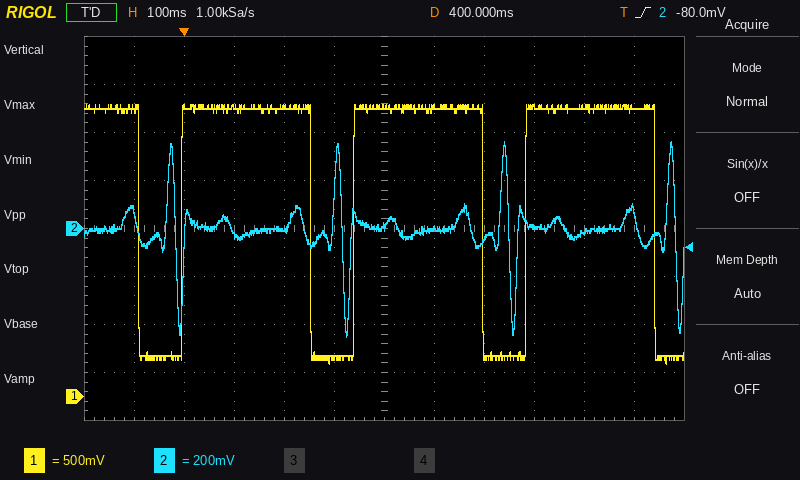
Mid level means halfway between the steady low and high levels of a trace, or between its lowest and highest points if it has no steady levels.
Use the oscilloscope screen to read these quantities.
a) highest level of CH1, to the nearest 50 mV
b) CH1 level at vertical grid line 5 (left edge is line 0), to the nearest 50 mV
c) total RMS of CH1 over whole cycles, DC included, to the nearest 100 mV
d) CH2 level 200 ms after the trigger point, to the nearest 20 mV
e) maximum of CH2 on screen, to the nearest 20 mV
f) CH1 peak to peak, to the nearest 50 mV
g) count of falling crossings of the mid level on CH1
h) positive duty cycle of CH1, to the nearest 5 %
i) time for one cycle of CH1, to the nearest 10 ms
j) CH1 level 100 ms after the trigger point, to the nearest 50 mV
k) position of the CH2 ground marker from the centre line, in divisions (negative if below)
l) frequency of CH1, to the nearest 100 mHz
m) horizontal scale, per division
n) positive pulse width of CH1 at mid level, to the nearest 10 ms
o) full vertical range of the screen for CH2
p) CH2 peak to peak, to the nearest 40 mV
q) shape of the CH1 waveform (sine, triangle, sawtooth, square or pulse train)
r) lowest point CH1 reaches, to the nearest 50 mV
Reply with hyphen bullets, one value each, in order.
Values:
- 3.05 V
- 400 mV
- 2.6 V
- 0 mV
- 360 mV
- 2.70 V
- 4
- 75 %
- 340 ms
- 3.00 V
- 0.0 div
- 2.9 Hz
- 100 ms
- 260 ms
- 1.6 V
- 800 mV
- pulse train
- 350 mV
